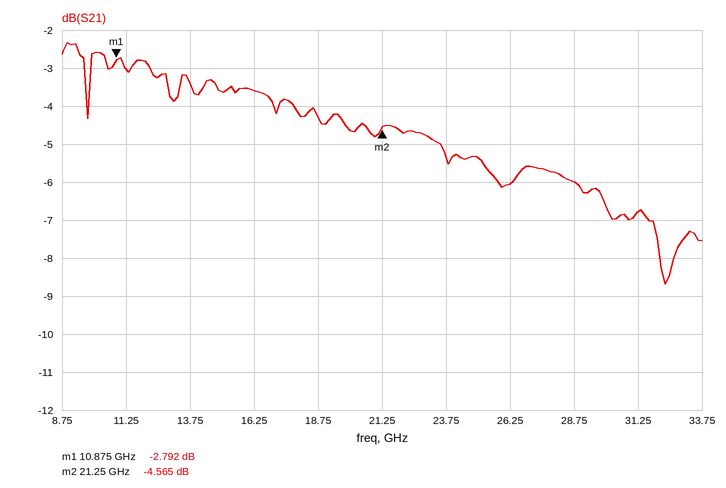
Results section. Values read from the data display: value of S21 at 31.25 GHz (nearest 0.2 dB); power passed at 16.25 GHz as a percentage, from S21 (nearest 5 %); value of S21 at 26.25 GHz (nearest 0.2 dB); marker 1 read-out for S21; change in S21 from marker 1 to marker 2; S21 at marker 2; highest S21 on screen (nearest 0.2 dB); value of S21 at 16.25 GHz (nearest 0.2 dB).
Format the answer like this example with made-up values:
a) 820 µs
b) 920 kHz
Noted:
a) -6.8 dB
b) 45 %
c) -6.0 dB
d) -2.792 dB
e) -1.773 dB
f) -4.565 dB
g) -2.4 dB
h) -3.6 dB
